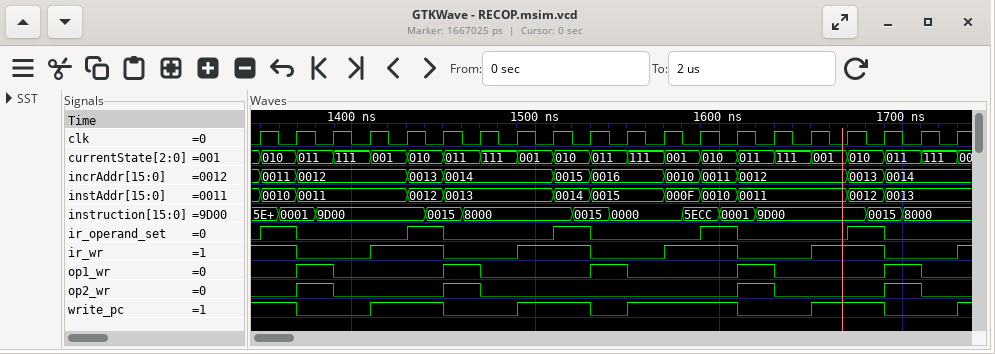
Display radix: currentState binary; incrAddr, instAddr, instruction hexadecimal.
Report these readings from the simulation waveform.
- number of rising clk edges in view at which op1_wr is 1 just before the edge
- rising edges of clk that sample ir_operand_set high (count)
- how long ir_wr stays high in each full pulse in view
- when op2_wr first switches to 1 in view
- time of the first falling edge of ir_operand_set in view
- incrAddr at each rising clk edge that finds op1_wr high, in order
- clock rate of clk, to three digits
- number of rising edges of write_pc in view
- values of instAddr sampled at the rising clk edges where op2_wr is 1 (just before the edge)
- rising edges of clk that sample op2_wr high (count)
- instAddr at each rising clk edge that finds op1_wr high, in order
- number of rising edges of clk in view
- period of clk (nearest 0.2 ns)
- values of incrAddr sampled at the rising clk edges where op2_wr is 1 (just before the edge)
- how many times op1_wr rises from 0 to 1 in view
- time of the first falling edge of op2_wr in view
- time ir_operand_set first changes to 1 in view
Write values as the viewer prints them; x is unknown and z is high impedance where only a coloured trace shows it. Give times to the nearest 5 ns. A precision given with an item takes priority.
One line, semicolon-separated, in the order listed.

5; 5; 40 ns, 40 ns, 40 ns, 40 ns; 1370 ns; 1370 ns; 0012, 0014, 0016, 0012, 0014; 50.0 MHz; 5; 0011, 0013, 0011, 0013; 4; 0011, 0013, 0015, 0011, 0013; 20; 20 ns; 0012, 0014, 0012, 0014; 5; 1390 ns; 1350 ns
